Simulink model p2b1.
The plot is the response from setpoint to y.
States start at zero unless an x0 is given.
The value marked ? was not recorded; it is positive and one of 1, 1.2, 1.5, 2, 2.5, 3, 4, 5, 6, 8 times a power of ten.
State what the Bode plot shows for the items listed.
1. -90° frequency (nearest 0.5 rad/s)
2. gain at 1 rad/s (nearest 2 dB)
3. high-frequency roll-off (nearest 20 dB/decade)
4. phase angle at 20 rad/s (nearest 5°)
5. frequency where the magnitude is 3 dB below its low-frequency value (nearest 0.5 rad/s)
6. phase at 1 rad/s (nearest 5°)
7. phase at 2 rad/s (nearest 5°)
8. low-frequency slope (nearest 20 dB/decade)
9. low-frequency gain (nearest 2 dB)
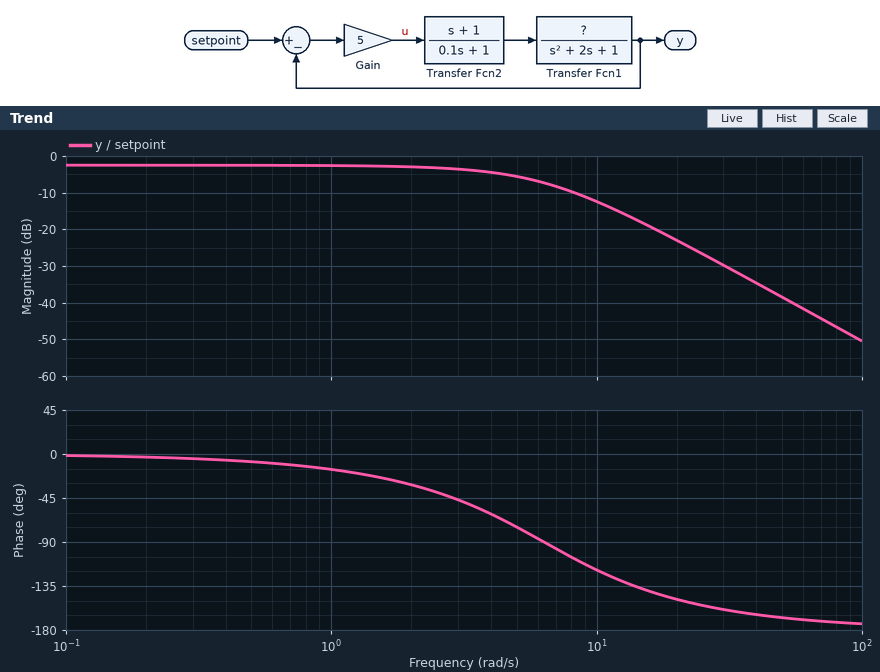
6.5 rad/s
-2 dB
-40 dB/decade
-150°
5.0 rad/s
-15°
-30°
0 dB/decade
-2 dB
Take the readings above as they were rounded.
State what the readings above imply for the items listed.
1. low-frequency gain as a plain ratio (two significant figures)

0.79
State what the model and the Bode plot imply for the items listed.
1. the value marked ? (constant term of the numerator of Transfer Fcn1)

0.6
